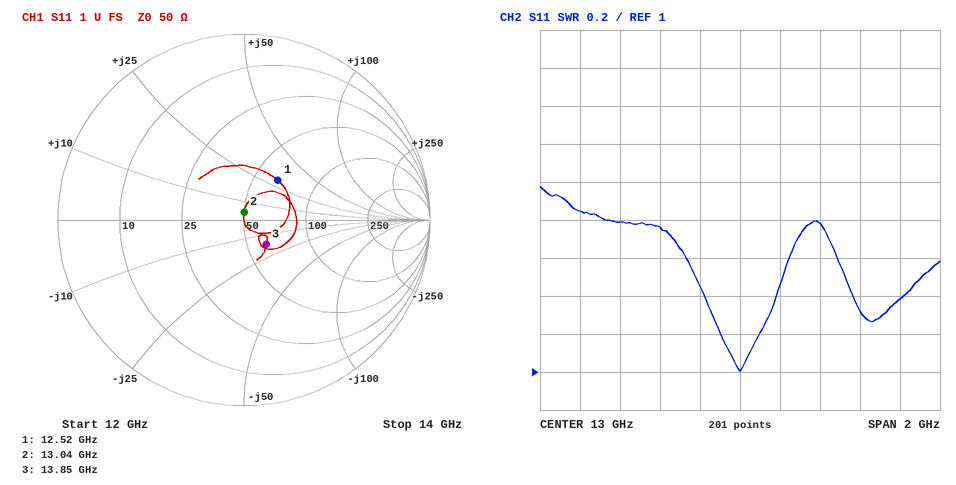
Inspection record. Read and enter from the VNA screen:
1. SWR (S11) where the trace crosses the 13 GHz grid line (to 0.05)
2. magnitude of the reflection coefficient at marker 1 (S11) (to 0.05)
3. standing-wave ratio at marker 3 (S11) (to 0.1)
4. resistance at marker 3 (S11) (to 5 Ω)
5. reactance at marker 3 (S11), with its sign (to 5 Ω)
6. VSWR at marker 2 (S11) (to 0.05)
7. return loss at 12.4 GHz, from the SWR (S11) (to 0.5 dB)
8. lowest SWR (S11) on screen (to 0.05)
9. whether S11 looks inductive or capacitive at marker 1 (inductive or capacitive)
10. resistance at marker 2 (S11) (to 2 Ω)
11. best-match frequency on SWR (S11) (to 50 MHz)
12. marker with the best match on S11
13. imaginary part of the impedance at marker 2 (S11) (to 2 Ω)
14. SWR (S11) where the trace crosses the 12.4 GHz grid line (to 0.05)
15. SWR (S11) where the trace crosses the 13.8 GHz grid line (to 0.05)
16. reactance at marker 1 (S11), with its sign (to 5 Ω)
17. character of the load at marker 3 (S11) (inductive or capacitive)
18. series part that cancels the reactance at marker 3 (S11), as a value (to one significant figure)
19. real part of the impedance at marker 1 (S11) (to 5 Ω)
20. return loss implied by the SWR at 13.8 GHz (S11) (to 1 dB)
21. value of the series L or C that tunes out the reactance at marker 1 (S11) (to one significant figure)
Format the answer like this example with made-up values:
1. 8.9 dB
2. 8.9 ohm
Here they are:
1. 1.00
2. 0.30
3. 1.4
4. 60 Ω
5. -15 Ω
6. 1.10
7. 11.0 dB
8. 1.00
9. inductive
10. 50 Ω
11. 13.00 GHz
12. marker 2
13. +4 Ω
14. 1.80
15. 1.40
16. +30 Ω
17. capacitive
18. 200 pH
19. 65 Ω
20. 16 dB
21. 400 fF
